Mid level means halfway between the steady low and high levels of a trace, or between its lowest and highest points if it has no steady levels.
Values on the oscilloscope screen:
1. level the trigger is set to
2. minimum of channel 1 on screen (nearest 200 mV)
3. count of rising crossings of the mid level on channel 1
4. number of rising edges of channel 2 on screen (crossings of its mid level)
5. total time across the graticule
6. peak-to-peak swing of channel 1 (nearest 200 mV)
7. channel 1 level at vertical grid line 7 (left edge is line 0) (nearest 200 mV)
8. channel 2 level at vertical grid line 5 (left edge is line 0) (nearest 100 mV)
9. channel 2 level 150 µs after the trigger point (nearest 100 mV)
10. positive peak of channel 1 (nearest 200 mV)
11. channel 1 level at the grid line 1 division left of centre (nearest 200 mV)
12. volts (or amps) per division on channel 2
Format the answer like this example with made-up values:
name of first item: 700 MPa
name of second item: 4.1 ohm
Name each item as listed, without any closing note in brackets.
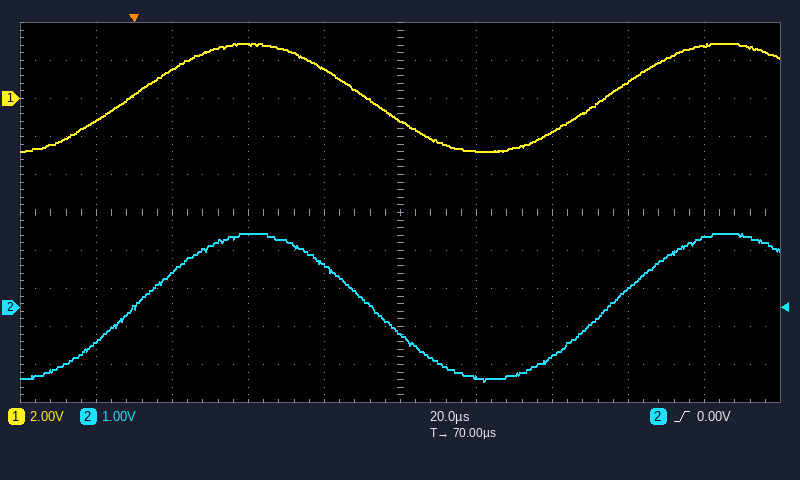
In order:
level the trigger is set to: 0.00 V
minimum of channel 1 on screen: -2.8 V
count of rising crossings of the mid level on channel 1: 2
number of rising edges of channel 2 on screen: 2
total time across the graticule: 200 µs
peak-to-peak swing of channel 1: 5.6 V
channel 1 level at vertical grid line 7 (left edge is line 0): -1.8 V
channel 2 level at vertical grid line 5 (left edge is line 0): -700 mV
channel 2 level 150 µs after the trigger point: 1.8 V
positive peak of channel 1: 2.8 V
channel 1 level at the grid line 1 division left of centre: 1.6 V
volts (or amps) per division on channel 2: 1 V
